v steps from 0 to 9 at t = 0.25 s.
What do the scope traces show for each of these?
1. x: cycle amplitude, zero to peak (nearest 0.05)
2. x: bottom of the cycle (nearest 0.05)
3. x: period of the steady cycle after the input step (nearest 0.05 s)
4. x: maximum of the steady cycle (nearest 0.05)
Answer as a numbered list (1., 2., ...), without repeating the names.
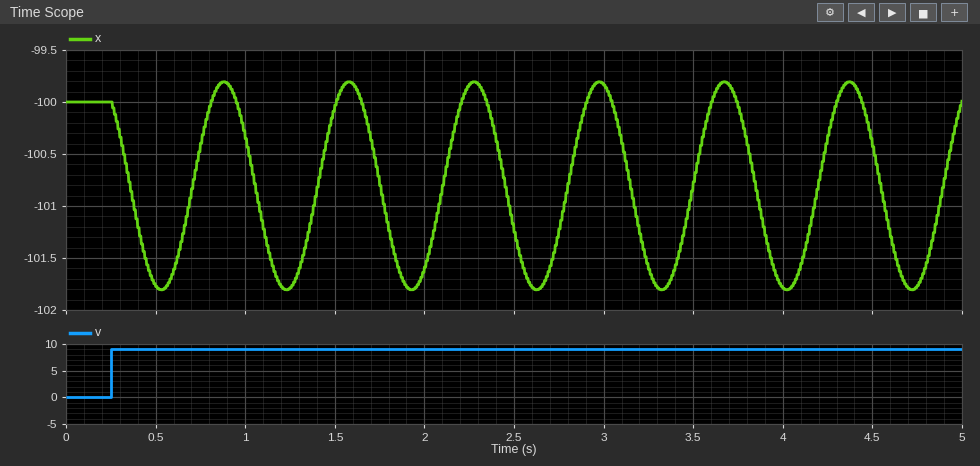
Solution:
1. 1.00
2. -101.80
3. 0.70 s
4. -99.80
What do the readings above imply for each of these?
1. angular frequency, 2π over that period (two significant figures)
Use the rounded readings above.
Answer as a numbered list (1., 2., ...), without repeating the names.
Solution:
1. 9.0 rad/s
